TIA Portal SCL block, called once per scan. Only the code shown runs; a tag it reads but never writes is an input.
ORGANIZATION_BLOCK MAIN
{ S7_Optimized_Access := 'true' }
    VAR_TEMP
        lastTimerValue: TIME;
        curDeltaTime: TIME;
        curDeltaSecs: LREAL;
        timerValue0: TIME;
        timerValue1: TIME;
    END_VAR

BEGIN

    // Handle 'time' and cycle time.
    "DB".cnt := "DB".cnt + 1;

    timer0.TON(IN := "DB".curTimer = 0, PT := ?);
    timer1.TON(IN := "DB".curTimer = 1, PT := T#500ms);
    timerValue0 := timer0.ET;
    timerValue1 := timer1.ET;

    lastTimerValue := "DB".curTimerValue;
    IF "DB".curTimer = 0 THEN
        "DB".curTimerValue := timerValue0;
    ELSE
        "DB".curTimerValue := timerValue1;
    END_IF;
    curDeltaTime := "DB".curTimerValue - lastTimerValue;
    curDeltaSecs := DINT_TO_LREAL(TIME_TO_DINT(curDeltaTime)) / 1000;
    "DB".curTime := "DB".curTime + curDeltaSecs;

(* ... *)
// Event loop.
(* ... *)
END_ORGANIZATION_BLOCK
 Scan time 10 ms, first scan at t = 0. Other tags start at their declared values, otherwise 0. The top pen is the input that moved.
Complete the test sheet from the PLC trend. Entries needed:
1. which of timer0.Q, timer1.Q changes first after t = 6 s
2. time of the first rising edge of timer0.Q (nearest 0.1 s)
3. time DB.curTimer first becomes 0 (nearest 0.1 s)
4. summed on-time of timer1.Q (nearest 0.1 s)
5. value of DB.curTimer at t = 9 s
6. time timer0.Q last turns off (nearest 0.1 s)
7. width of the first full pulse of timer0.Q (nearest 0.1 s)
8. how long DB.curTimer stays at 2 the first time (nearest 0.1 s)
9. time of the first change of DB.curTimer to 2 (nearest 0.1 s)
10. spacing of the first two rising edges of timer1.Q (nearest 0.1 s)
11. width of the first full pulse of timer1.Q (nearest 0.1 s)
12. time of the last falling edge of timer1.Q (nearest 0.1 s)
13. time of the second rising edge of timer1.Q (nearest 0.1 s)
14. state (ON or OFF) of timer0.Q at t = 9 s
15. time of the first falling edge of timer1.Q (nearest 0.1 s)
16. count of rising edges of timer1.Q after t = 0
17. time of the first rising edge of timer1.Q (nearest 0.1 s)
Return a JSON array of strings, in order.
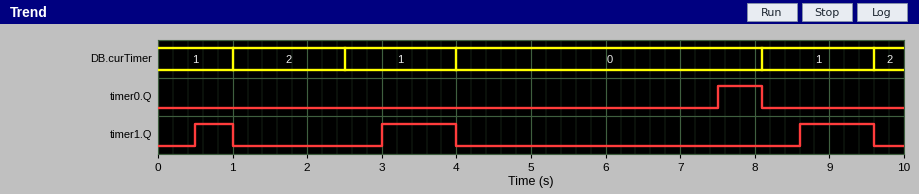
["timer0.Q", "7.5 s", "4.0 s", "2.5 s", "1", "8.1 s", "0.6 s", "1.5 s", "1.0 s", "2.5 s", "0.5 s", "9.6 s", "3.0 s", "OFF", "1.0 s", "3", "0.5 s"]
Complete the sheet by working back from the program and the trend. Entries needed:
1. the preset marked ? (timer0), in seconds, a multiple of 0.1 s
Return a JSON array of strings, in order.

["3.5 s"]
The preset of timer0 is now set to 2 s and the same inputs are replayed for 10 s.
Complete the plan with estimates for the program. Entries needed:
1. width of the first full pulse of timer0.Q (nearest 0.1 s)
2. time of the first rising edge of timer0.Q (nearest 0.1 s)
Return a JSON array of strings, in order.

["2.1 s", "6.0 s"]
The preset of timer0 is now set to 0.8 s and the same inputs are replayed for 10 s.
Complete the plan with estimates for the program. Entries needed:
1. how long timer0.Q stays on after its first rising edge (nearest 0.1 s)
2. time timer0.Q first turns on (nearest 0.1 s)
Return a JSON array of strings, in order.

["3.3 s", "4.8 s"]
